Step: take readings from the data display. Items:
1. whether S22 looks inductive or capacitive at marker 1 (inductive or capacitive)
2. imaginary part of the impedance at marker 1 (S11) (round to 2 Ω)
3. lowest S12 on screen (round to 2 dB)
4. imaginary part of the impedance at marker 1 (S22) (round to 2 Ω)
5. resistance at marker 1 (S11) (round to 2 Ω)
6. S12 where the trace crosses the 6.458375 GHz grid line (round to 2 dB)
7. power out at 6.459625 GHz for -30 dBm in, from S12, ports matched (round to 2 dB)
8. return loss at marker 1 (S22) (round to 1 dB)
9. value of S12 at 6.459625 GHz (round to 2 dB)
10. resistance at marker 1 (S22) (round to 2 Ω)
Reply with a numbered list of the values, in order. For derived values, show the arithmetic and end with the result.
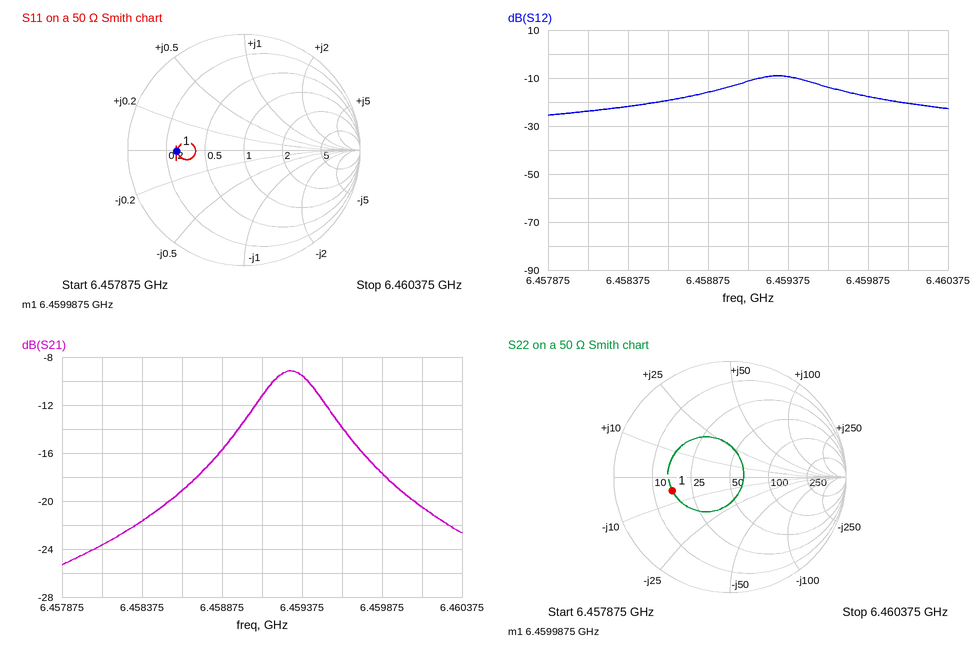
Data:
1. capacitive
2. 0 Ω
3. -26 dB
4. -6 Ω
5. 14 Ω
6. -22 dB
7. -30 dBm + (-14 dB) = -44 dBm
8. 6 dB
9. -14 dB
10. 16 Ω
